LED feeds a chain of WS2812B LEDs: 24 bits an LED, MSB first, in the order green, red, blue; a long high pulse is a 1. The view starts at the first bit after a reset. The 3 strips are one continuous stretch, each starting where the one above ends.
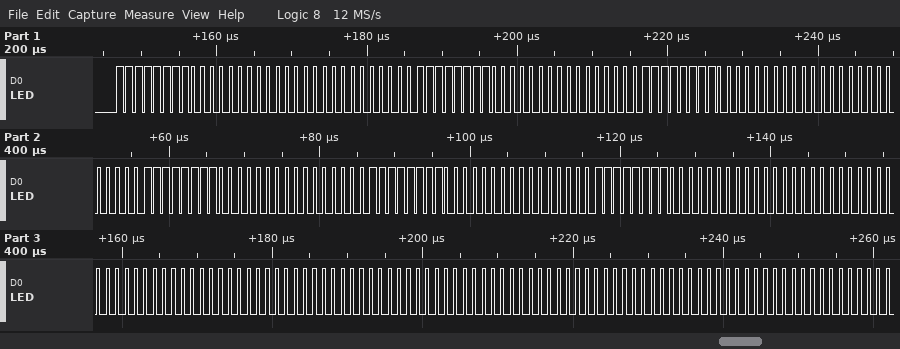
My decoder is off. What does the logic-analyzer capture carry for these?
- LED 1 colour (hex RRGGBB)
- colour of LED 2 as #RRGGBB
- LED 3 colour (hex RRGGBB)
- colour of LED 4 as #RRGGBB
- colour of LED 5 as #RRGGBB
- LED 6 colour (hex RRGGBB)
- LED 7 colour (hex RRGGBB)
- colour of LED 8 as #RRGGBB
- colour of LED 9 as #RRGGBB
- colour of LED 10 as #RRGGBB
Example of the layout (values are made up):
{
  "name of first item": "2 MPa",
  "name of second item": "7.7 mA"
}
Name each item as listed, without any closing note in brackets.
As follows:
{
  "LED 1 colour": "#00FF00",
  "colour of LED 2 as #RRGGBB": "#FF0000",
  "LED 3 colour": "#FF0000",
  "colour of LED 4 as #RRGGBB": "#0000FF",
  "colour of LED 5 as #RRGGBB": "#0000FF",
  "LED 6 colour": "#0000FF",
  "LED 7 colour": "#000000",
  "colour of LED 8 as #RRGGBB": "#000000",
  "colour of LED 9 as #RRGGBB": "#000000",
  "colour of LED 10 as #RRGGBB": "#000000"
}
